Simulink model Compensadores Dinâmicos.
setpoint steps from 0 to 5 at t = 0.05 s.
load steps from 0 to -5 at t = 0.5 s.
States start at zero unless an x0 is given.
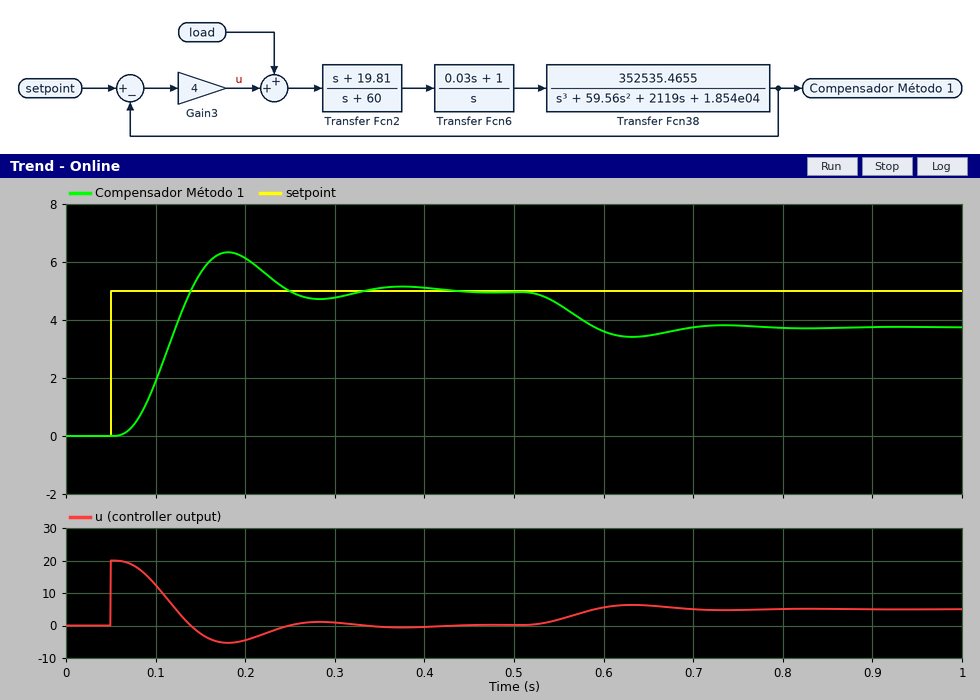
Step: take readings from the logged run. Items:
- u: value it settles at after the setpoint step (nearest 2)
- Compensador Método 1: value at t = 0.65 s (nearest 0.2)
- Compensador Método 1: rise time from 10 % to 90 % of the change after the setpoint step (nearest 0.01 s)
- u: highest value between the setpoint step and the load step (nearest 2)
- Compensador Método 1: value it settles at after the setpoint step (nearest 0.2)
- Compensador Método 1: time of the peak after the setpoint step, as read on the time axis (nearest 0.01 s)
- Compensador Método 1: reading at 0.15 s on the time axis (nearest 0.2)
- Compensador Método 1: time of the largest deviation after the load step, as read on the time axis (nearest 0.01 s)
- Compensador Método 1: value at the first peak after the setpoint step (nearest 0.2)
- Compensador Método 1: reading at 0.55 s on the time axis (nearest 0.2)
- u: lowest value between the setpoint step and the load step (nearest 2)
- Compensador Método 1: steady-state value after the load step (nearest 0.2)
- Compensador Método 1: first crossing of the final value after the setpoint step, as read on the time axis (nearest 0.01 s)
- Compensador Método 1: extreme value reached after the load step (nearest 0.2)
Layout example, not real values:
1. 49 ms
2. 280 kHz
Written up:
1. 0
2. 3.4
3. 0.05 s
4. 20
5. 5.0
6. 0.18 s
7. 5.6
8. 0.63 s
9. 6.4
10. 4.6
11. -6
12. 3.8
13. 0.14 s
14. 3.4
